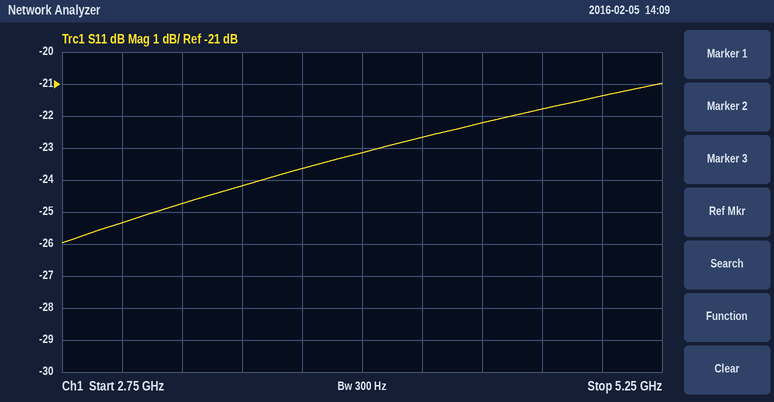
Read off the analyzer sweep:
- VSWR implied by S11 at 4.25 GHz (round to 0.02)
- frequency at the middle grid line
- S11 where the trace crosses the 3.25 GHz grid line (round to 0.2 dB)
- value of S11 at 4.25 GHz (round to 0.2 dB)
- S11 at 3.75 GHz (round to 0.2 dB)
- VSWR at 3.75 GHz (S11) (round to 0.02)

1.16
4 GHz
-24.8 dB
-22.6 dB
-23.6 dB
1.14
